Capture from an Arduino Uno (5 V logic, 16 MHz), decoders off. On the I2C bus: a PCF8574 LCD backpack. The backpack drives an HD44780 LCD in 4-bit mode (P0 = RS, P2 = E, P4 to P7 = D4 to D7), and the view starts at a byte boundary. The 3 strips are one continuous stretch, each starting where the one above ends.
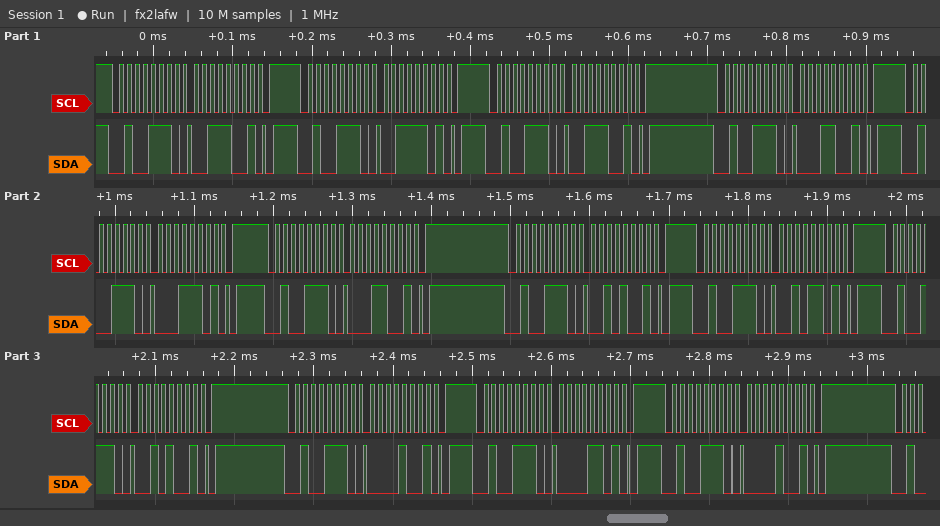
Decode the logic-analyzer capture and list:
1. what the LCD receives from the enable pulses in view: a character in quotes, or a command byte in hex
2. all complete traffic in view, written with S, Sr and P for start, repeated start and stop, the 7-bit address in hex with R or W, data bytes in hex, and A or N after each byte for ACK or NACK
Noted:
'1' ' '
S 27W A 39 A P S 27W A 3D A P S 27W A 39 A P S 27W A 19 A P S 27W A 1D A P S 27W A 19 A P S 27W A 29 A P S 27W A 2D A P S 27W A 29 A P S 27W A 09 A P S 27W A 0D A P S 27W A 09 A P
